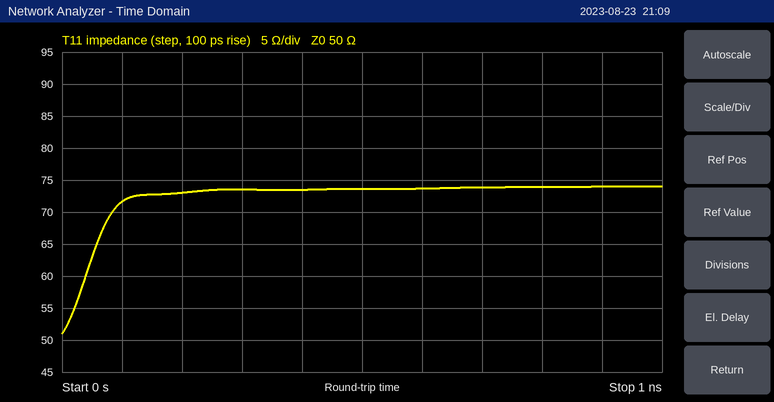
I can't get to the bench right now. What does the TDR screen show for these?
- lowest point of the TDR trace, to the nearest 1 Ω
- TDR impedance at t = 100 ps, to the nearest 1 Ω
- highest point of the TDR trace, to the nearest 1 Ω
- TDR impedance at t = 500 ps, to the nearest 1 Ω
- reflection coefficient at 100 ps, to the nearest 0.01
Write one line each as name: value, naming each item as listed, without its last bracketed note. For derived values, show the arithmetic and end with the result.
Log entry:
lowest point of the TDR trace, to the nearest 1 Ω: 51 Ω
TDR impedance at t = 100 ps, to the nearest 1 Ω: 72 Ω
highest point of the TDR trace, to the nearest 1 Ω: 74 Ω
TDR impedance at t = 500 ps, to the nearest 1 Ω: 74 Ω
reflection coefficient at 100 ps, to the nearest 0.01: (72 − 50)/(72 + 50) ≈ +0.18
